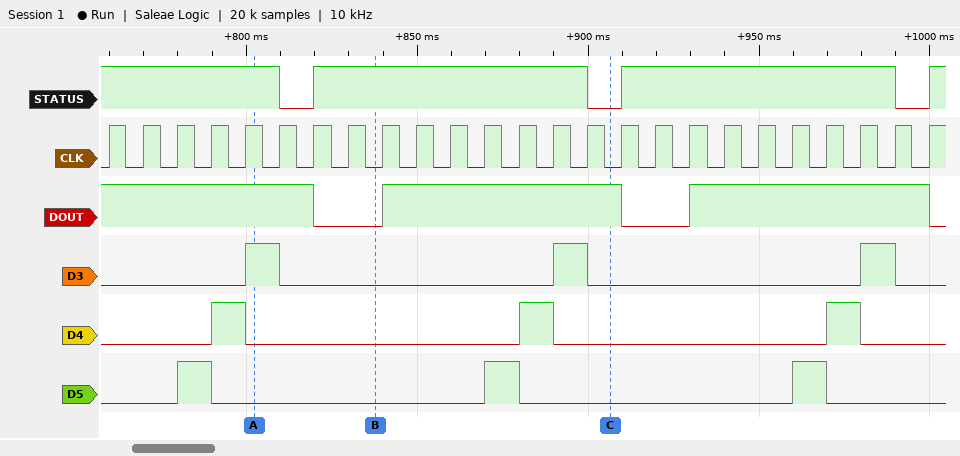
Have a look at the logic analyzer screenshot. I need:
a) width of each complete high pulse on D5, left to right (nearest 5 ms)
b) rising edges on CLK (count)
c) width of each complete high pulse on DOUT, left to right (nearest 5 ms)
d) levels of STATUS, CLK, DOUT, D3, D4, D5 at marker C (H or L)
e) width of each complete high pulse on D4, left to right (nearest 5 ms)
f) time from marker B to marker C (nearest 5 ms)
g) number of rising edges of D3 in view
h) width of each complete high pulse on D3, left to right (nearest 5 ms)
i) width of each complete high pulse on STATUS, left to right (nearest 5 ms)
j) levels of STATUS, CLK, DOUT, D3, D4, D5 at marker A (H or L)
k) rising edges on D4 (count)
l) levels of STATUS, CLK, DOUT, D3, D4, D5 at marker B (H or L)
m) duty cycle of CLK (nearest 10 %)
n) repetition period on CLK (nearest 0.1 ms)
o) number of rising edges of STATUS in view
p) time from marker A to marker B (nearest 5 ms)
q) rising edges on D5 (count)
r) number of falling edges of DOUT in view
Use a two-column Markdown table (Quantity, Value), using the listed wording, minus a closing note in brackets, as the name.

| Quantity | Value |
|---|---|
| width of each complete high pulse on D5, left to right | 10 ms, 10 ms, 10 ms |
| rising edges on CLK | 25 |
| width of each complete high pulse on DOUT, left to right | 70 ms, 70 ms |
| levels of STATUS, CLK, DOUT, D3, D4, D5 at marker C | STATUS=L, CLK=L, DOUT=H, D3=L, D4=L, D5=L |
| width of each complete high pulse on D4, left to right | 10 ms, 10 ms, 10 ms |
| time from marker B to marker C | 70 ms |
| number of rising edges of D3 in view | 3 |
| width of each complete high pulse on D3, left to right | 10 ms, 10 ms, 10 ms |
| width of each complete high pulse on STATUS, left to right | 80 ms, 80 ms |
| levels of STATUS, CLK, DOUT, D3, D4, D5 at marker A | STATUS=H, CLK=H, DOUT=H, D3=H, D4=L, D5=L |
| rising edges on D4 | 3 |
| levels of STATUS, CLK, DOUT, D3, D4, D5 at marker B | STATUS=H, CLK=L, DOUT=L, D3=L, D4=L, D5=L |
| duty cycle of CLK | 50 % |
| repetition period on CLK | 10 ms |
| number of rising edges of STATUS in view | 3 |
| time from marker A to marker B | 35 ms |
| rising edges on D5 | 3 |
| number of falling edges of DOUT in view | 3 |
